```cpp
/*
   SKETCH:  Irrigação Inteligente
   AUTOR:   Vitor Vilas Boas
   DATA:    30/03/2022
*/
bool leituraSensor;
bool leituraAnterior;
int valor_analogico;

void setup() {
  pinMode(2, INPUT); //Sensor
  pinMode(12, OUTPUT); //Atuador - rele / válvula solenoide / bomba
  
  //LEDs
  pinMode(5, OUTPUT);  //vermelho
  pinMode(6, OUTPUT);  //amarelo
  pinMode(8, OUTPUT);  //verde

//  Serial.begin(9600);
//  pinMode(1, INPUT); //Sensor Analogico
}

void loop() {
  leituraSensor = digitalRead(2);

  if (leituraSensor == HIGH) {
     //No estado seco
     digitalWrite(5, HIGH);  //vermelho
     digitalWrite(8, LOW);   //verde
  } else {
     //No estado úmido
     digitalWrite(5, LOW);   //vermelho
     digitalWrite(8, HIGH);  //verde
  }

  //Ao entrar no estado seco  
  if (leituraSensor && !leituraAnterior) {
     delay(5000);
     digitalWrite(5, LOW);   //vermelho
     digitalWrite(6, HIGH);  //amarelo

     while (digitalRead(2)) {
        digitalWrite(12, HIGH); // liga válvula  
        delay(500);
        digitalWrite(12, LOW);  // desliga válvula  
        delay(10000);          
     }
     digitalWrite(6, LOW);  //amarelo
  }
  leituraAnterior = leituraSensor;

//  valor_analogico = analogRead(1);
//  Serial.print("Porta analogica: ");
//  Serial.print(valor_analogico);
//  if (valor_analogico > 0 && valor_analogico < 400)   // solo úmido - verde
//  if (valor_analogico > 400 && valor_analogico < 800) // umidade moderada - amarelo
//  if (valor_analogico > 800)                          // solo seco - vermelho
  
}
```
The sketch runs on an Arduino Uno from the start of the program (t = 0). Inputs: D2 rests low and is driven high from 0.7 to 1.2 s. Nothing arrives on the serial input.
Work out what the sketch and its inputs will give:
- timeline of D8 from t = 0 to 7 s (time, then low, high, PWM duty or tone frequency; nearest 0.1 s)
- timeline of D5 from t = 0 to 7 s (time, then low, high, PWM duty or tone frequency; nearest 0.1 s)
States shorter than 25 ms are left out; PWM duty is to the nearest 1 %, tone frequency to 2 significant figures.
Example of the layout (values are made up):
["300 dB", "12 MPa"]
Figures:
["0 s high; 0.7 s low; 5.7 s high", "0 s low; 0.7 s high; 5.7 s low"]
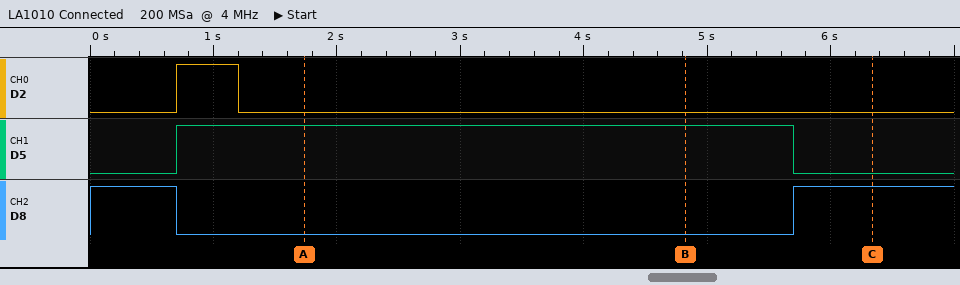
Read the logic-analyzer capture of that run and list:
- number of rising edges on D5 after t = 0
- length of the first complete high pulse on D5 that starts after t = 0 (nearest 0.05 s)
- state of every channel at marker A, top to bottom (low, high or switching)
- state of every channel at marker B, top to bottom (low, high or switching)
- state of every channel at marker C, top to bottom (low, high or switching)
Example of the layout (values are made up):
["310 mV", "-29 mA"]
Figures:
["1", "5.00 s", "D2 low, D5 high, D8 low", "D2 low, D5 high, D8 low", "D2 low, D5 low, D8 high"]
